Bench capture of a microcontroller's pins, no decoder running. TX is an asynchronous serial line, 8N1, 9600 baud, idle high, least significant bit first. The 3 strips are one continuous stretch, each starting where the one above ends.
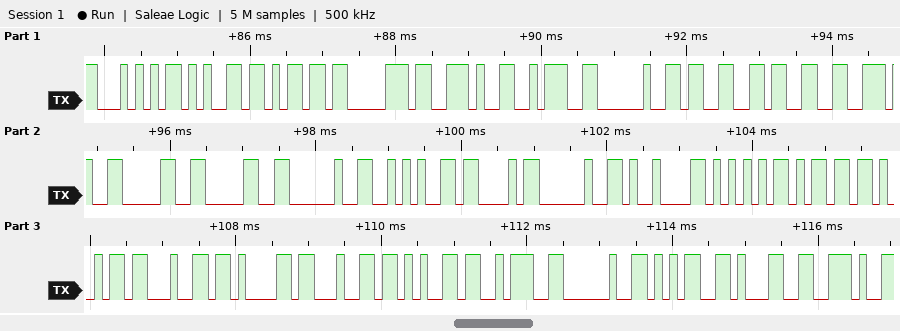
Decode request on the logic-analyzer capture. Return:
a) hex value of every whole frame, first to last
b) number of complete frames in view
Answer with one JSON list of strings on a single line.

["54 65 6D 70 2E 3A 20 33 33 2E 30 30 20 2A 43 20 09 55 6D 69 64 61 64 65 3A 20 35 31 2E", "29"]
